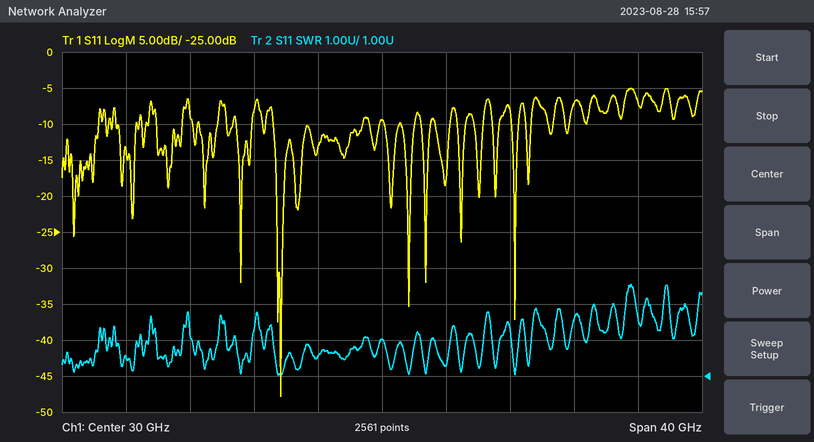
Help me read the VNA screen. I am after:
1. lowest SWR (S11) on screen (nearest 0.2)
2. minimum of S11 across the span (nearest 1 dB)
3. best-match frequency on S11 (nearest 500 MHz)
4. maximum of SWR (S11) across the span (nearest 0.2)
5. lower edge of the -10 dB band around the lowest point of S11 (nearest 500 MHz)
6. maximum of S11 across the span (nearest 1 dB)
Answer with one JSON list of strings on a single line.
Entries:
["1.0", "-48 dB", "23.5 GHz", "3.6", "23.0 GHz", "-5 dB"]
